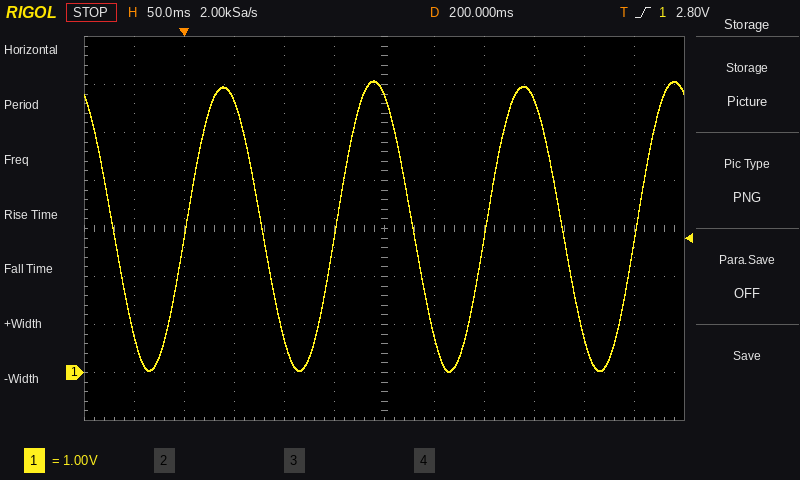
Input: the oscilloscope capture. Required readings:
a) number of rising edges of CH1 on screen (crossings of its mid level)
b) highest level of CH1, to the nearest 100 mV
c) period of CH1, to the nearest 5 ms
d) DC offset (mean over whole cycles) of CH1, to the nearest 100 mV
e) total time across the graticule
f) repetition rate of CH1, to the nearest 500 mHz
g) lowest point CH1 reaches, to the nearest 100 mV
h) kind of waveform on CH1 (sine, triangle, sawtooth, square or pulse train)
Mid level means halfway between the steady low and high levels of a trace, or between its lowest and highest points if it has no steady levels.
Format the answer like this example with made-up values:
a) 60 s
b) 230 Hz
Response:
a) 4
b) 6.1 V
c) 150 ms
d) 3.1 V
e) 600 ms
f) 6.5 Hz
g) 0.0 V
h) sine
